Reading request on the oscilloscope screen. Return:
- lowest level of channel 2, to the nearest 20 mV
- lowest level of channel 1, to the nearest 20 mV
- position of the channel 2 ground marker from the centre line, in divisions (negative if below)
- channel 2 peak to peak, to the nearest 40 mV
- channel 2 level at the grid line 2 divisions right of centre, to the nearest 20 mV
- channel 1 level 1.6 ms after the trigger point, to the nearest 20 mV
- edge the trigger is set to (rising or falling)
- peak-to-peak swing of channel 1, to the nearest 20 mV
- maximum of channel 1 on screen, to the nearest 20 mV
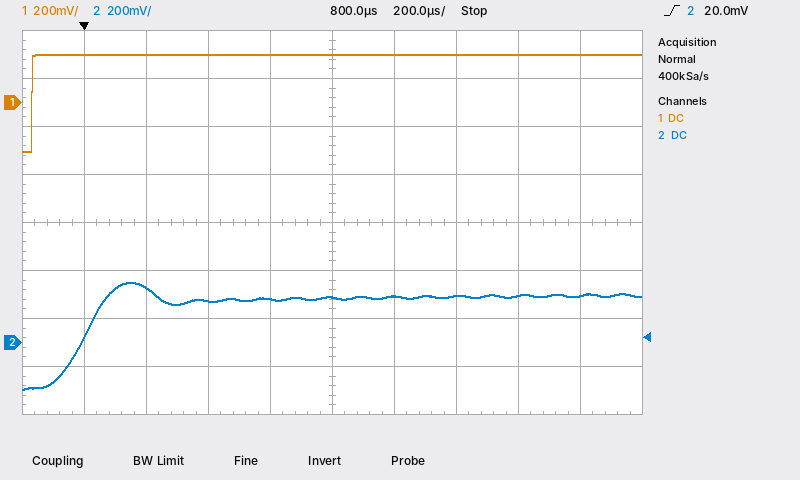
-200 mV
-200 mV
-2.5 div
440 mV
200 mV
200 mV
rising
400 mV
200 mV
